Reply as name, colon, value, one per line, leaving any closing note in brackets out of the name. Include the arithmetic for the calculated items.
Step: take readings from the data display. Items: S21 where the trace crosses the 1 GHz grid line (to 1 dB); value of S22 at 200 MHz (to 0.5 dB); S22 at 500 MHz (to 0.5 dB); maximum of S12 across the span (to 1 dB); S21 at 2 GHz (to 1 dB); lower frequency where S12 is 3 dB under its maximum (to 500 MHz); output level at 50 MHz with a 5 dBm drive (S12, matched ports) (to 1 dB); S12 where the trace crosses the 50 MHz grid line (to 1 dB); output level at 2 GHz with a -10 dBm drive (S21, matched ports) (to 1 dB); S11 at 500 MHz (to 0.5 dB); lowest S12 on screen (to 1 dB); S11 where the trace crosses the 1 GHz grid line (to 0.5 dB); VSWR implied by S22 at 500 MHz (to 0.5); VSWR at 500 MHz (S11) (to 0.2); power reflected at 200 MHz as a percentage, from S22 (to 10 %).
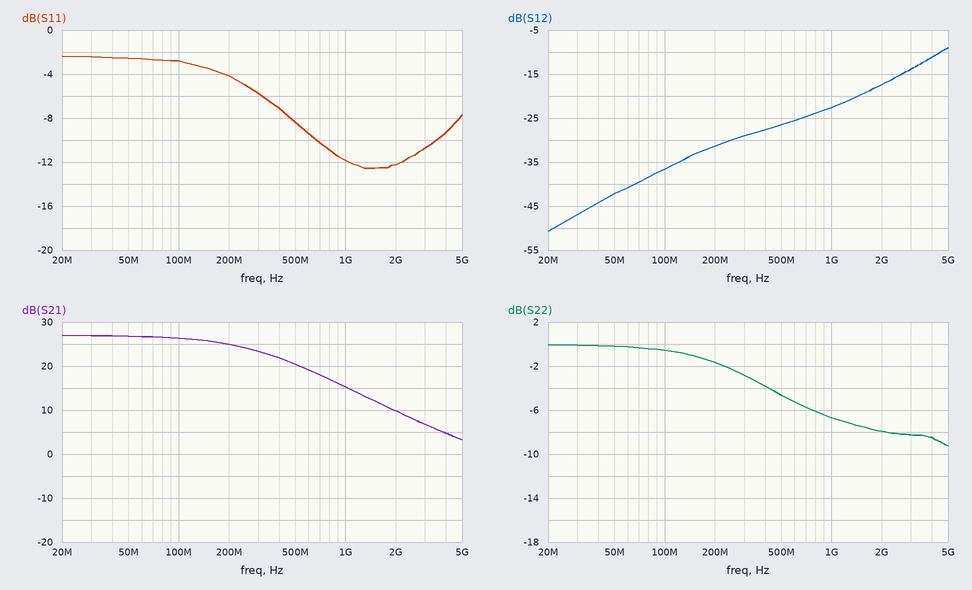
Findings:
S21 where the trace crosses the 1 GHz grid line: 15 dB
value of S22 at 200 MHz: -1.5 dB
S22 at 500 MHz: -4.5 dB
maximum of S12 across the span: -9 dB
S21 at 2 GHz: 10 dB
lower frequency where S12 is 3 dB under its maximum: 3.5 GHz
output level at 50 MHz with a 5 dBm drive (S12, matched ports): 5 dBm + (-42 dB) = -37 dBm
S12 where the trace crosses the 50 MHz grid line: -42 dB
output level at 2 GHz with a -10 dBm drive (S21, matched ports): -10 dBm + (10 dB) = 0 dBm
S11 at 500 MHz: -8.5 dB
lowest S12 on screen: -51 dB
S11 where the trace crosses the 1 GHz grid line: -12.0 dB
VSWR implied by S22 at 500 MHz: |Γ| = 10^(-4.5/20) = 0.5957; VSWR = (1 + 0.5957)/(1 − 0.5957) ≈ 4.0
VSWR at 500 MHz (S11): |Γ| = 10^(-8.5/20) = 0.3758; VSWR = (1 + 0.3758)/(1 − 0.3758) ≈ 2.2
power reflected at 200 MHz as a percentage, from S22: 10^(-1.5/10) ≈ 70.8 %, so 70 % to the nearest 10 %
